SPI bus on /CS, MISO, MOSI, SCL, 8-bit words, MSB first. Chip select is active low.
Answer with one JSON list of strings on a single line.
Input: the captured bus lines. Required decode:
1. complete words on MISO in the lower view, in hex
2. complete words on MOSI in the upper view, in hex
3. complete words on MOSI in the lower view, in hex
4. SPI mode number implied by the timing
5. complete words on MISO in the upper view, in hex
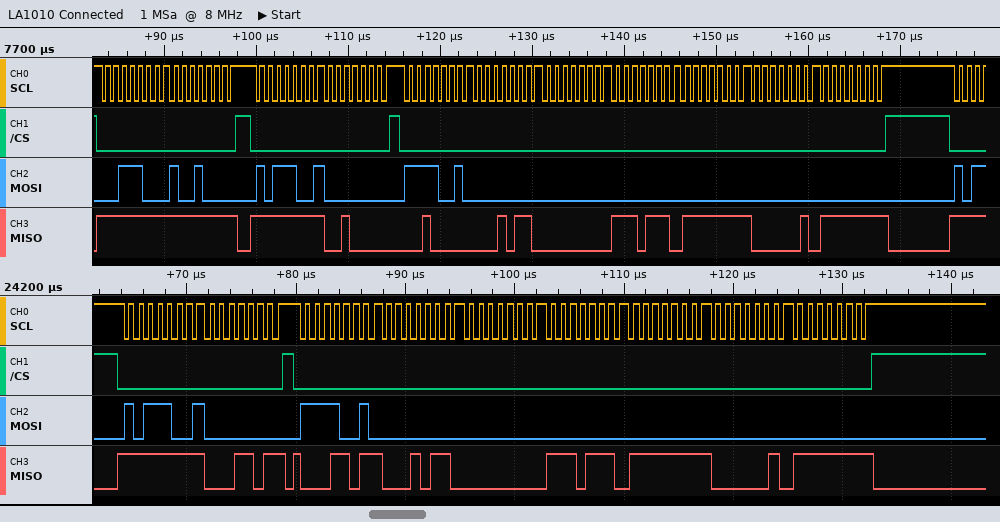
["FF, 1B, 1B, 16, 00, EE, FF, 02, FF", "38, 90, B9, 00, F2, 00, 00, 00, 00, 00, 00", "B9, 00, F2, 00, 00, 00, 00, 00, 00", "3", "FF, FF, FF, 20, 20, 16, 00, EE, FF, 02, FF"]
